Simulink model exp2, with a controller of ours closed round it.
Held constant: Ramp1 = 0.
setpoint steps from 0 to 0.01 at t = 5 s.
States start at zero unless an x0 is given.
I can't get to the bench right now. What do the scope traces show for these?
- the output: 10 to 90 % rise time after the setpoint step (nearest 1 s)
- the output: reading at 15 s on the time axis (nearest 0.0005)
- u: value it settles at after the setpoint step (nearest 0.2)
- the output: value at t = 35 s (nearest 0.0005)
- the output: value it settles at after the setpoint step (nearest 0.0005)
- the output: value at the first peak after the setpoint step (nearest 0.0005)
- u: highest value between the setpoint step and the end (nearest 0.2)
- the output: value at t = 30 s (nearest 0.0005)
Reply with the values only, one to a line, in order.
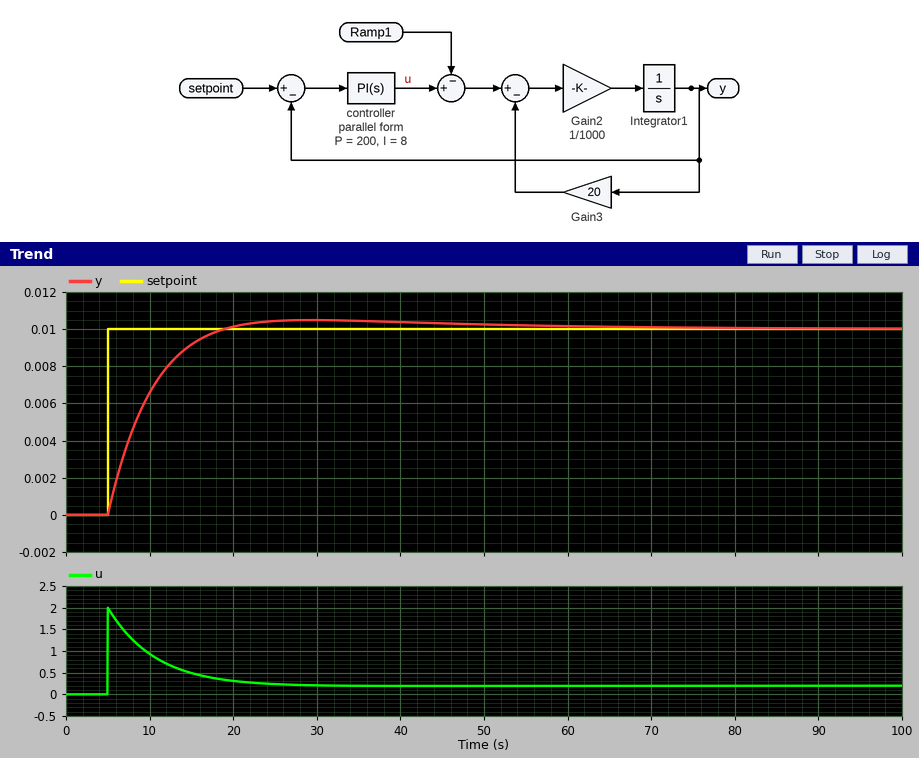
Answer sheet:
9 s
0.0090
0.2
0.0105
0.0100
0.0105
2.0
0.0105
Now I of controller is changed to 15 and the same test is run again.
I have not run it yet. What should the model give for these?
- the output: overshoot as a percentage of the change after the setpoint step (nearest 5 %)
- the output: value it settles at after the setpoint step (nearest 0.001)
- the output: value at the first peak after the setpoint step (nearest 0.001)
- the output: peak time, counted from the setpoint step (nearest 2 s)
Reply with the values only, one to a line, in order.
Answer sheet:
10 %
0.010
0.011
18 s
